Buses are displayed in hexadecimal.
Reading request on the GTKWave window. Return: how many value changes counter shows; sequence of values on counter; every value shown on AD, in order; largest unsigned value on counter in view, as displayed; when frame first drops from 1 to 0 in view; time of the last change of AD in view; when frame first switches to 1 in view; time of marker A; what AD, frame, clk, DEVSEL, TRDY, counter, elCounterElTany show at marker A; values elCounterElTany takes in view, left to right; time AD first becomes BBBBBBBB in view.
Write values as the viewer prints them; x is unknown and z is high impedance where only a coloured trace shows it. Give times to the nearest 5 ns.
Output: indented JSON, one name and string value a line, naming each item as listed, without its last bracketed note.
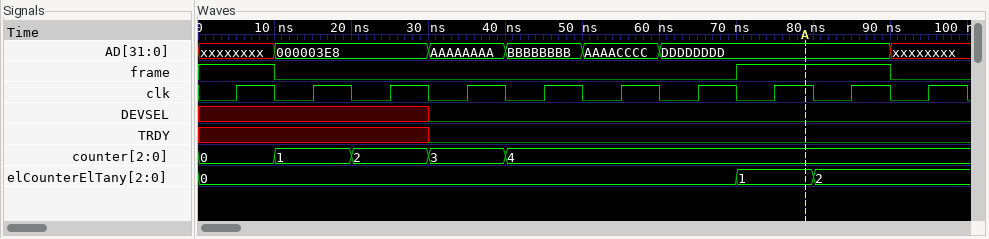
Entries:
{
  "how many value changes counter shows": "4",
  "sequence of values on counter": "0, 1, 2, 3, 4",
  "every value shown on AD, in order": "xxxxxxxx, 000003E8, AAAAAAAA, BBBBBBBB, AAAACCCC, DDDDDDDD, xxxxxxxx",
  "largest unsigned value on counter in view, as displayed": "4",
  "when frame first drops from 1 to 0 in view": "10 ns",
  "time of the last change of AD in view": "90 ns",
  "when frame first switches to 1 in view": "70 ns",
  "time of marker A": "80 ns",
  "what AD, frame, clk, DEVSEL, TRDY, counter, elCounterElTany show at marker A": "AD=DDDDDDDD, frame=1, clk=1, DEVSEL=0, TRDY=0, counter=4, elCounterElTany=1",
  "values elCounterElTany takes in view, left to right": "0, 1, 2",
  "time AD first becomes BBBBBBBB in view": "40 ns"
}
